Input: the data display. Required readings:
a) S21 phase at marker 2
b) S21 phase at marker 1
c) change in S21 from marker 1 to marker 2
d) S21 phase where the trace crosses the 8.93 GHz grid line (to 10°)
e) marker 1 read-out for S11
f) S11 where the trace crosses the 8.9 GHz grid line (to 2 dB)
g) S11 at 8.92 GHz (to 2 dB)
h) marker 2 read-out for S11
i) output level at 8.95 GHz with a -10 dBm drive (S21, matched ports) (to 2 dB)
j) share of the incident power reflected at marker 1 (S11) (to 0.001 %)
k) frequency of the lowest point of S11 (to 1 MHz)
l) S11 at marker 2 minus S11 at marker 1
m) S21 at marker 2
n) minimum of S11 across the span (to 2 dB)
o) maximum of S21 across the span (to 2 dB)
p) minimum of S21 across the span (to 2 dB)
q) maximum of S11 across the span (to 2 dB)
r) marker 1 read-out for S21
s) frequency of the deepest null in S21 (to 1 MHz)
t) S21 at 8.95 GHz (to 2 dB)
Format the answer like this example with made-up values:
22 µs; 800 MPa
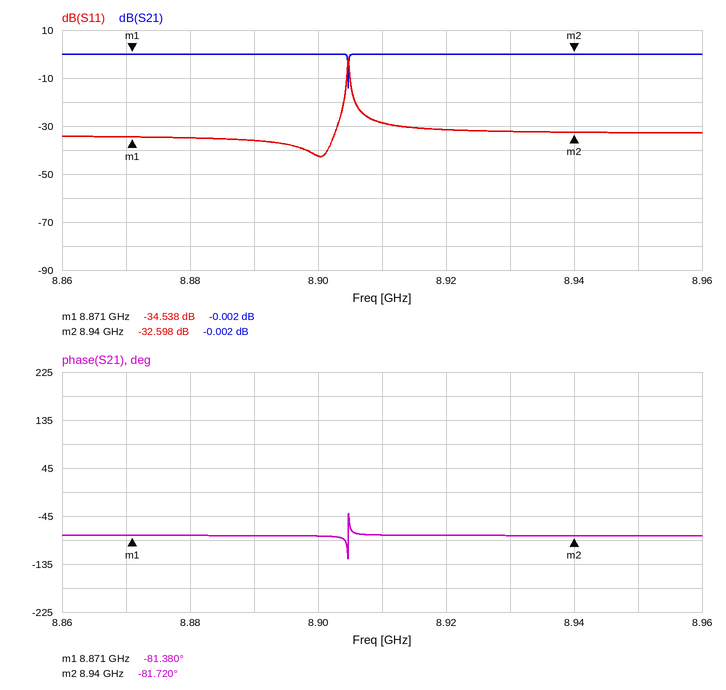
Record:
-81.720°; -81.380°; 0.000 dB; -80°; -34.538 dB; -42 dB; -32 dB; -32.598 dB; -10 dBm; 0.035 %; 8.900 GHz; 1.940 dB; -0.002 dB; -42 dB; 0 dB; -14 dB; -2 dB; -0.002 dB; 8.905 GHz; 0 dB
